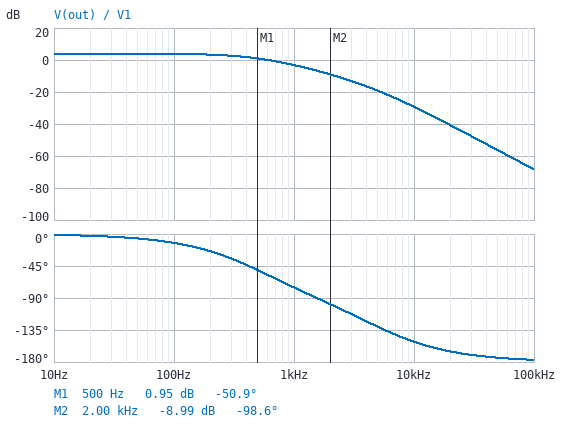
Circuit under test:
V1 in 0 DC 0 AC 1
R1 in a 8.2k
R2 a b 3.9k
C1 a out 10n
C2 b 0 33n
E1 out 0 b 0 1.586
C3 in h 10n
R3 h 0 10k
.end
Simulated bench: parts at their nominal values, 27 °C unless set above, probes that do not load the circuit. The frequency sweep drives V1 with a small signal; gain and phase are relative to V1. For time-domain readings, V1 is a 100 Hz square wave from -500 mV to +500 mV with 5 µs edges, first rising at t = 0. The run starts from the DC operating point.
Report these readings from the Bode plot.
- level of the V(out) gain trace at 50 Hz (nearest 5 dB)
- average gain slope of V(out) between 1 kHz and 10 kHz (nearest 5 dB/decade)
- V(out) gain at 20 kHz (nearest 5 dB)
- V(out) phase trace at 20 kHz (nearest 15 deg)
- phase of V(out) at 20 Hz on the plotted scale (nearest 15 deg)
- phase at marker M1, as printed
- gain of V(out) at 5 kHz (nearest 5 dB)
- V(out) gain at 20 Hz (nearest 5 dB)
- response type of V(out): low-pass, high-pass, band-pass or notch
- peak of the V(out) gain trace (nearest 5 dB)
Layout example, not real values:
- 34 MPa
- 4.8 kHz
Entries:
- 5 dB
- -25 dB/decade
- -40 dB
- -165 deg
- 0 deg
- -50.9 deg
- -20 dB
- 5 dB
- low-pass
- 5 dB
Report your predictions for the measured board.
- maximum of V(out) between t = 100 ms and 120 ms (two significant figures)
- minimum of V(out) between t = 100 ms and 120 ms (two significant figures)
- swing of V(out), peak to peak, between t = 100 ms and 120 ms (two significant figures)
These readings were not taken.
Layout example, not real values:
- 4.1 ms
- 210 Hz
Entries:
- 790 mV
- -790 mV
- 1.6 V
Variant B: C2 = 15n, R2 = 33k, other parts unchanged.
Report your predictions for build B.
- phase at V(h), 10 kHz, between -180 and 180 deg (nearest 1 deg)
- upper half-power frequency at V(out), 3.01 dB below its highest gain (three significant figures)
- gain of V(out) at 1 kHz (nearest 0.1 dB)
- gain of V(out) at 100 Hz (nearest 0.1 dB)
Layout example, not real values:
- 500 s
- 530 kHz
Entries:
- 9 deg
- 318 Hz
- -7.2 dB
- 3.6 dB
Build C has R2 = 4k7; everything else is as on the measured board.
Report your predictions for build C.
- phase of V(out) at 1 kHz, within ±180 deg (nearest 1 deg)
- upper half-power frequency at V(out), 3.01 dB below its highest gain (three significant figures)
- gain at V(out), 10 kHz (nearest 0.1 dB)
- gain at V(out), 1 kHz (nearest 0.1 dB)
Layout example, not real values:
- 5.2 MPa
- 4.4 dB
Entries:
- -78 deg
- 462 Hz
- -30.7 dB
- -3.7 dB
